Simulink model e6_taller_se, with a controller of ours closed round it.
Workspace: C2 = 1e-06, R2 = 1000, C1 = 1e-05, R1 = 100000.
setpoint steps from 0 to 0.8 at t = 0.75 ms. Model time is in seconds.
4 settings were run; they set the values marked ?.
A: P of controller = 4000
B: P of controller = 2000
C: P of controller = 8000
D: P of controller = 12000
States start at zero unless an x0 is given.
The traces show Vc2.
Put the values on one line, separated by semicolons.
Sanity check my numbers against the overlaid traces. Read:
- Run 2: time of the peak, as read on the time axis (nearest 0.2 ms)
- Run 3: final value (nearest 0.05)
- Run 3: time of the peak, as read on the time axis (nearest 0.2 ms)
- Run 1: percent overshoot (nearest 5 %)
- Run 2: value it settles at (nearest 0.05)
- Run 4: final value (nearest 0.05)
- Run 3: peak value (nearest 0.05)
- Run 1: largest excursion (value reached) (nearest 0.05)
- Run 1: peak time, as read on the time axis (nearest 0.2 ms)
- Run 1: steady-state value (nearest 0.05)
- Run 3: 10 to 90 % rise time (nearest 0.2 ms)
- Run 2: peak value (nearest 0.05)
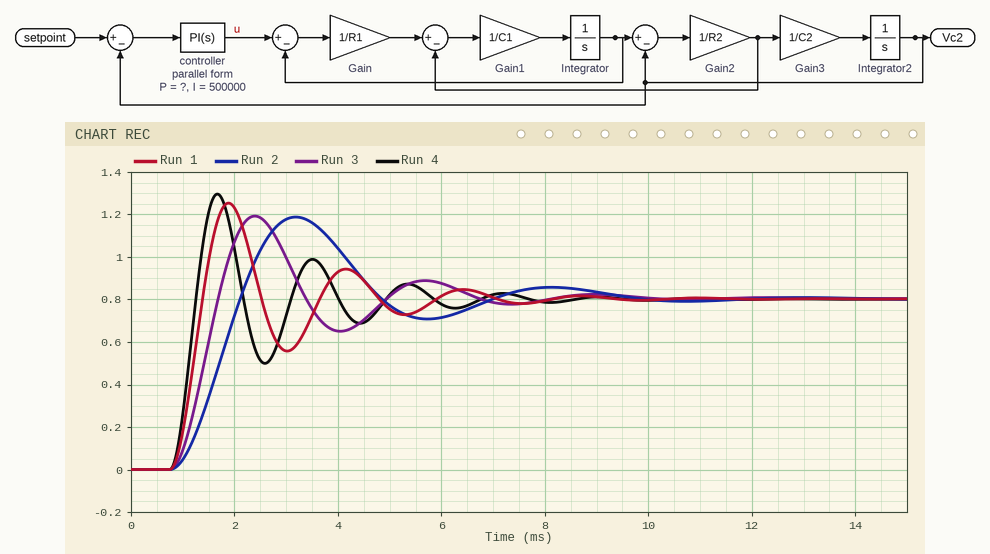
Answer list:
3.2 ms; 0.80; 2.4 ms; 55 %; 0.80; 0.80; 1.20; 1.25; 1.8 ms; 0.80; 0.6 ms; 1.20
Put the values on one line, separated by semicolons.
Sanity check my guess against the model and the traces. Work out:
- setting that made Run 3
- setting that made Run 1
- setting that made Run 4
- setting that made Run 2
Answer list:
A; C; D; B
